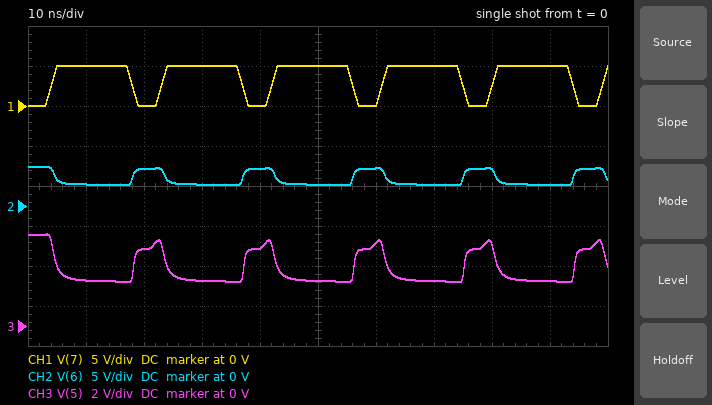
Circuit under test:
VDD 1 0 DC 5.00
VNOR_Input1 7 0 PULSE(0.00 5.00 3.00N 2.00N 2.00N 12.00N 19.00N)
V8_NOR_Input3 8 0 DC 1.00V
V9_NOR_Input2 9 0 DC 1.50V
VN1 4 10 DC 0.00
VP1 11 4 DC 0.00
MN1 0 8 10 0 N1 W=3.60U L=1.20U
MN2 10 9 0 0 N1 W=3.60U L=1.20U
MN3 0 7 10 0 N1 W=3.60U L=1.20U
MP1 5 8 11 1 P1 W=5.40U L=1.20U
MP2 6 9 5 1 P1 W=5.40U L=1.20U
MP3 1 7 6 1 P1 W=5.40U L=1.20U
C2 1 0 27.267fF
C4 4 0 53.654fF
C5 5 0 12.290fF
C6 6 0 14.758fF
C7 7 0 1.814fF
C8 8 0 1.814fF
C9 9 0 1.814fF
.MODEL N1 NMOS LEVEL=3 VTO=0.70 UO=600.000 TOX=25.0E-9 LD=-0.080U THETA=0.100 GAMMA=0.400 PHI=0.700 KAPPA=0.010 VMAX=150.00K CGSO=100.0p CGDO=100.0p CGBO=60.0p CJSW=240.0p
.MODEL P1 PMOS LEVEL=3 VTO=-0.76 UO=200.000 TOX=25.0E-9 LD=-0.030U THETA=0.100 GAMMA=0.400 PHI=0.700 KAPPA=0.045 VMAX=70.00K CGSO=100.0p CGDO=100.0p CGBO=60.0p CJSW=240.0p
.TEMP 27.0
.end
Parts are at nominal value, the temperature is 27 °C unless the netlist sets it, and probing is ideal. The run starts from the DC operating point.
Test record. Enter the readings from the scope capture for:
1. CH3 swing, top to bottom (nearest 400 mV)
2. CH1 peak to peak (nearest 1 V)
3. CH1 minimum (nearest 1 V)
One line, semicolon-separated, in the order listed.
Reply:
2.4 V; 5 V; 0 V
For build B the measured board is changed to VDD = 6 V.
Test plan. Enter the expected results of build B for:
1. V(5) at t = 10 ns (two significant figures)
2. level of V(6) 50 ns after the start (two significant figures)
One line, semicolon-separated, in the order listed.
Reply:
2.5 V; 2.9 V
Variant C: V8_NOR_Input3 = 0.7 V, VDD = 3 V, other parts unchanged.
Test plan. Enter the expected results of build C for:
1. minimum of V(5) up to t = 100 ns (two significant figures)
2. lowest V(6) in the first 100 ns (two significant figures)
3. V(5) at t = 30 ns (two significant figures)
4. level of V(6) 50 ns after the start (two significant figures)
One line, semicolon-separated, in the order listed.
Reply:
1.7 V; 2.3 V; 1.8 V; 2.4 V
